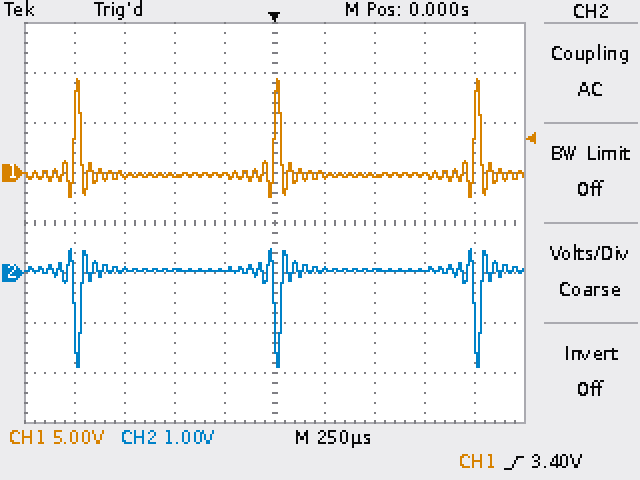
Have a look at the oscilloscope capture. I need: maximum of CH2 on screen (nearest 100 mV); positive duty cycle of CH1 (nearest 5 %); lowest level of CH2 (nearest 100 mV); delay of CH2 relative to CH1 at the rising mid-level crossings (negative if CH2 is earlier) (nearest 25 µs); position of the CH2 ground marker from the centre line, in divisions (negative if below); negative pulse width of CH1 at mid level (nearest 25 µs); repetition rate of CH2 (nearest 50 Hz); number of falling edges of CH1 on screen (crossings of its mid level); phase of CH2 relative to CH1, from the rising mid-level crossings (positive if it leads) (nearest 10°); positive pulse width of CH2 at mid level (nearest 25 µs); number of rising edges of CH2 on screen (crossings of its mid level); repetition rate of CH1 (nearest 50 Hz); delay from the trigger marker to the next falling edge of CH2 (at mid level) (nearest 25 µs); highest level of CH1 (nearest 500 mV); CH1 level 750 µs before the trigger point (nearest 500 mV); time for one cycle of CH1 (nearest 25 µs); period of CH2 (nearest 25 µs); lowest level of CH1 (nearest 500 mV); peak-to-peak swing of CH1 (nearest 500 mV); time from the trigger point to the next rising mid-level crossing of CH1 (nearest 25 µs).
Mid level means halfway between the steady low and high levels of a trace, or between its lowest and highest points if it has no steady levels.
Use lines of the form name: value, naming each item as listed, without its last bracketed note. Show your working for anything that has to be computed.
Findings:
maximum of CH2 on screen: 500 mV
positive duty cycle of CH1: 5 %
lowest level of CH2: -1.9 V
delay of CH2 relative to CH1 at the rising mid-level crossings (negative if CH2 is earlier): +25 µs
position of the CH2 ground marker from the centre line, in divisions: -1.0 div
negative pulse width of CH1 at mid level: 975 µs
repetition rate of CH2: 1 / 1.000 ms ≈ 1.00 kHz
number of falling edges of CH1 on screen: 3
phase of CH2 relative to CH1, from the rising mid-level crossings (positive if it leads): −360° × (+25 µs) / 1.000 ms ≈ -9.00°, so -10° to the nearest 10°
positive pulse width of CH2 at mid level: 975 µs
number of rising edges of CH2 on screen: 3
repetition rate of CH1: 1 / 1.000 ms ≈ 1.00 kHz
delay from the trigger marker to the next falling edge of CH2 (at mid level): 1.000 ms
highest level of CH1: 9.5 V
CH1 level 750 µs before the trigger point: 0.0 V
time for one cycle of CH1: 1.000 ms
period of CH2: 1.000 ms
lowest level of CH1: -2.5 V
peak-to-peak swing of CH1: 9.5 V − (-2.5 V) = 12.0 V
time from the trigger point to the next rising mid-level crossing of CH1: 1.000 ms
